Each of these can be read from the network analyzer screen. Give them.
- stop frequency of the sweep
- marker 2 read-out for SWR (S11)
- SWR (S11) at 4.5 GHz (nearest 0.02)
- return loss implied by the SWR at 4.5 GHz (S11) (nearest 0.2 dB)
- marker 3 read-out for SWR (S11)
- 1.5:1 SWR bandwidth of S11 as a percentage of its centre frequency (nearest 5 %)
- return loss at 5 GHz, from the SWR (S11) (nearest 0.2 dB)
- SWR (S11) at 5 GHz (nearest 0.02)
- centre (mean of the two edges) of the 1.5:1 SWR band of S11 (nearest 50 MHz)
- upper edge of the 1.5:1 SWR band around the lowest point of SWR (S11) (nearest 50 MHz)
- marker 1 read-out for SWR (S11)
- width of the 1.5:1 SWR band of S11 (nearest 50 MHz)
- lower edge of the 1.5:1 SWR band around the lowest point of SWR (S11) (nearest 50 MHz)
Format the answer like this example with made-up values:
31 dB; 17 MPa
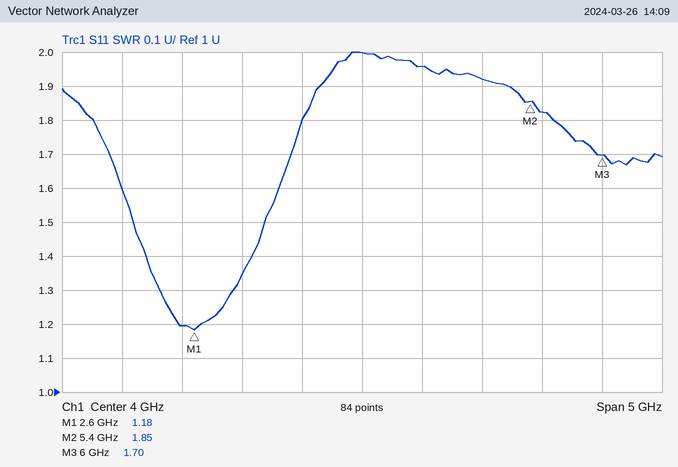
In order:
6.5 GHz; 1.85; 1.96; 9.8 dB; 1.70; 40 %; 10.0 dB; 1.92; 2.65 GHz; 3.20 GHz; 1.18; 1.10 GHz; 2.10 GHz
